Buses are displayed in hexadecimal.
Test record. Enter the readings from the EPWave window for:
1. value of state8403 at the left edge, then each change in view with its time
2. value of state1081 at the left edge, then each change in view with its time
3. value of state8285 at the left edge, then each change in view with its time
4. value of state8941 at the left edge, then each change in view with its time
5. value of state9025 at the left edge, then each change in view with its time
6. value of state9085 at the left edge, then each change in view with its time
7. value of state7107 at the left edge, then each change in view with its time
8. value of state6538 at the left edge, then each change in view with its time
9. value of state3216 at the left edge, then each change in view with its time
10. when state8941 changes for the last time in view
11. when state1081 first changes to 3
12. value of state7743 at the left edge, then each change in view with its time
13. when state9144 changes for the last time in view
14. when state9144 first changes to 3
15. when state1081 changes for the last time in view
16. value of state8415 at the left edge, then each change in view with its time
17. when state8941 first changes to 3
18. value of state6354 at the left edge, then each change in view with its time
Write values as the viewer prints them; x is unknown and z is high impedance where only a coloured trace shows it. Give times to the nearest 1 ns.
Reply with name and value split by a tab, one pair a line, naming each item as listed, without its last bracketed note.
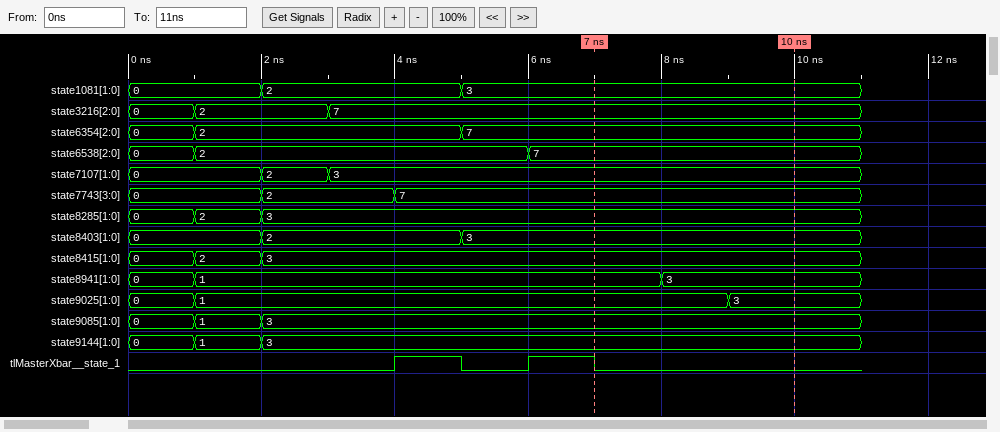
value of state8403 at the left edge, then each change in view with its time	0, 2 at 2 ns, 3 at 5 ns
value of state1081 at the left edge, then each change in view with its time	0, 2 at 2 ns, 3 at 5 ns
value of state8285 at the left edge, then each change in view with its time	0, 2 at 1 ns, 3 at 2 ns
value of state8941 at the left edge, then each change in view with its time	0, 1 at 1 ns, 3 at 8 ns
value of state9025 at the left edge, then each change in view with its time	0, 1 at 1 ns, 3 at 9 ns
value of state9085 at the left edge, then each change in view with its time	0, 1 at 1 ns, 3 at 2 ns
value of state7107 at the left edge, then each change in view with its time	0, 2 at 2 ns, 3 at 3 ns
value of state6538 at the left edge, then each change in view with its time	0, 2 at 1 ns, 7 at 6 ns
value of state3216 at the left edge, then each change in view with its time	0, 2 at 1 ns, 7 at 3 ns
when state8941 changes for the last time in view	8 ns
when state1081 first changes to 3	5 ns
value of state7743 at the left edge, then each change in view with its time	0, 2 at 2 ns, 7 at 4 ns
when state9144 changes for the last time in view	2 ns
when state9144 first changes to 3	2 ns
when state1081 changes for the last time in view	5 ns
value of state8415 at the left edge, then each change in view with its time	0, 2 at 1 ns, 3 at 2 ns
when state8941 first changes to 3	8 ns
value of state6354 at the left edge, then each change in view with its time	0, 2 at 1 ns, 7 at 5 ns
